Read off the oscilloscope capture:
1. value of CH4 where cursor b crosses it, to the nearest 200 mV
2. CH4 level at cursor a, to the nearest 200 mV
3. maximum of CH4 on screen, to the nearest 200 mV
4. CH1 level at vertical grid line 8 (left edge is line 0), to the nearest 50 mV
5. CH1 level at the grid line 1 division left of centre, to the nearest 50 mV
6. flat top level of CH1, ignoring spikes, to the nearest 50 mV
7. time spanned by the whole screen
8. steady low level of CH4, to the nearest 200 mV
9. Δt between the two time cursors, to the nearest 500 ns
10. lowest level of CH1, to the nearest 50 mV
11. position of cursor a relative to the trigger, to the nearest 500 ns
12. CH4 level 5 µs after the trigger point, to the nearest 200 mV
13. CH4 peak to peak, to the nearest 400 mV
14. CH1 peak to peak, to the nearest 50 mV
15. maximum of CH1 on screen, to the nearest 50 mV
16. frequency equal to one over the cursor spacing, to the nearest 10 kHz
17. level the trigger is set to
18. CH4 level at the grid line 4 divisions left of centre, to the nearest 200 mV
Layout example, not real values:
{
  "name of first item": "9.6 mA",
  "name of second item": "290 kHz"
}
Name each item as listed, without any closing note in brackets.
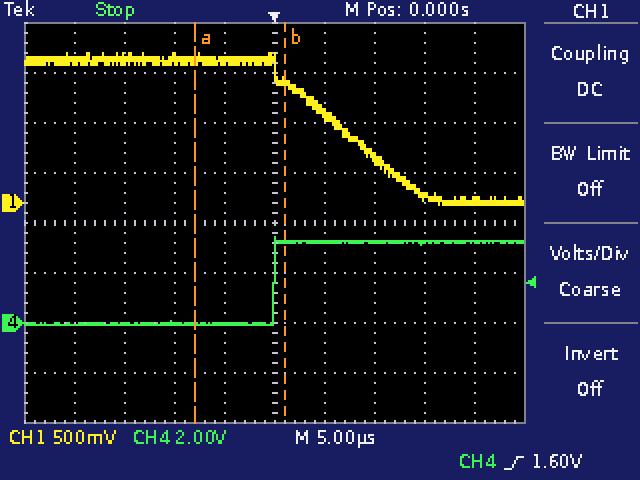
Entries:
{
  "value of CH4 where cursor b crosses it, to the nearest 200 mV": "3.2 V",
  "CH4 level at cursor a, to the nearest 200 mV": "0.0 V",
  "maximum of CH4 on screen, to the nearest 200 mV": "3.4 V",
  "CH1 level at vertical grid line 8 (left edge is line 0), to the nearest 50 mV": "50 mV",
  "CH1 level at the grid line 1 division left of centre, to the nearest 50 mV": "1.40 V",
  "flat top level of CH1, ignoring spikes, to the nearest 50 mV": "1.40 V",
  "time spanned by the whole screen": "50 µs",
  "steady low level of CH4, to the nearest 200 mV": "0.0 V",
  "Δt between the two time cursors, to the nearest 500 ns": "9.0 µs",
  "lowest level of CH1, to the nearest 50 mV": "0 mV",
  "position of cursor a relative to the trigger, to the nearest 500 ns": "-8.0 µs",
  "CH4 level 5 µs after the trigger point, to the nearest 200 mV": "3.2 V",
  "CH4 peak to peak, to the nearest 400 mV": "3.6 V",
  "CH1 peak to peak, to the nearest 50 mV": "1.50 V",
  "maximum of CH1 on screen, to the nearest 50 mV": "1.50 V",
  "frequency equal to one over the cursor spacing, to the nearest 10 kHz": "110 kHz",
  "level the trigger is set to": "1.60 V",
  "CH4 level at the grid line 4 divisions left of centre, to the nearest 200 mV": "0.0 V"
}
